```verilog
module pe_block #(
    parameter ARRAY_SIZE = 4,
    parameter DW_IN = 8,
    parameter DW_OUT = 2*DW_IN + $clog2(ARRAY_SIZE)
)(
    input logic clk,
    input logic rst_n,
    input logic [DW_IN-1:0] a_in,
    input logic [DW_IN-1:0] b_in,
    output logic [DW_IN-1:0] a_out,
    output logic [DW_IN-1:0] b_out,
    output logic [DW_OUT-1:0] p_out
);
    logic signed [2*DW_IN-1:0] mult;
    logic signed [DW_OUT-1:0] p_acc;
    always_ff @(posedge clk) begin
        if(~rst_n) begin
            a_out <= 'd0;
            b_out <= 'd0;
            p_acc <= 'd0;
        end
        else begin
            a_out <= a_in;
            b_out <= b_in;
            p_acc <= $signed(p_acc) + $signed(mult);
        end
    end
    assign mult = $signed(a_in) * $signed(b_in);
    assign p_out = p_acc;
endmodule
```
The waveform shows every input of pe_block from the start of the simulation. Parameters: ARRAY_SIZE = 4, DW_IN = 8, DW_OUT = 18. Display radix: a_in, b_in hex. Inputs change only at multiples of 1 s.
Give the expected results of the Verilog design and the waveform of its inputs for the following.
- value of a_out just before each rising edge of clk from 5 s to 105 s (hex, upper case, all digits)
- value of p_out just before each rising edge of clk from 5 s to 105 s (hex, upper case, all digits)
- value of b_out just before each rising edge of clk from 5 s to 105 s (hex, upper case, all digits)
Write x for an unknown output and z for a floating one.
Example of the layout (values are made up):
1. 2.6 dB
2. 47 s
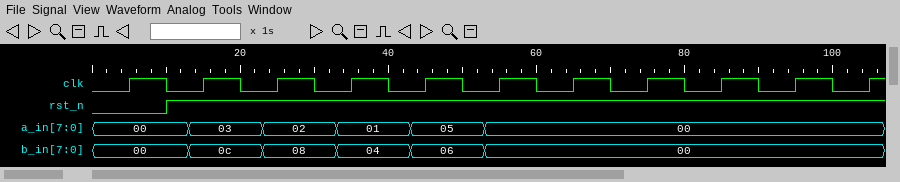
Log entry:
1. x, 00, 03, 02, 01, 05, 00, 00, 00, 00, 00
2. x, 00000, 00024, 00034, 00038, 00056, 00056, 00056, 00056, 00056, 00056
3. x, 00, 0C, 08, 04, 06, 00, 00, 00, 00, 00
